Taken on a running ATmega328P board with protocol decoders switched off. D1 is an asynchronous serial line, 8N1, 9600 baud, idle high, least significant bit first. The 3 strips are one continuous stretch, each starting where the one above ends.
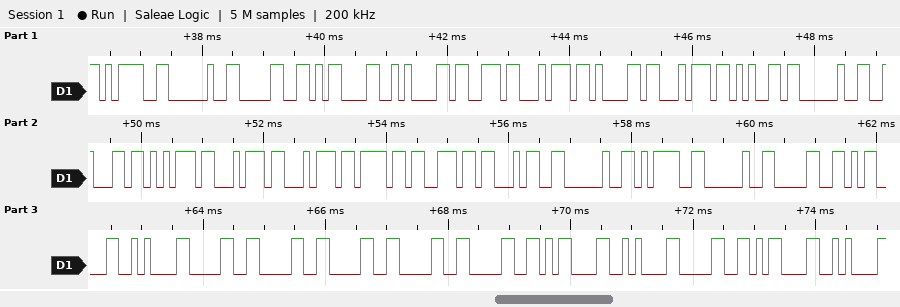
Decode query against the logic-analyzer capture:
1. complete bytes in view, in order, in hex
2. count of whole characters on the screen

3D 20 30 0D 0A 73 74 61 74 65 20 62 75 74 74 6F 6E 34 20 3D 20 30 0D 0A 30 30 30 30 30 0D 0A 30 0D 0A
34
